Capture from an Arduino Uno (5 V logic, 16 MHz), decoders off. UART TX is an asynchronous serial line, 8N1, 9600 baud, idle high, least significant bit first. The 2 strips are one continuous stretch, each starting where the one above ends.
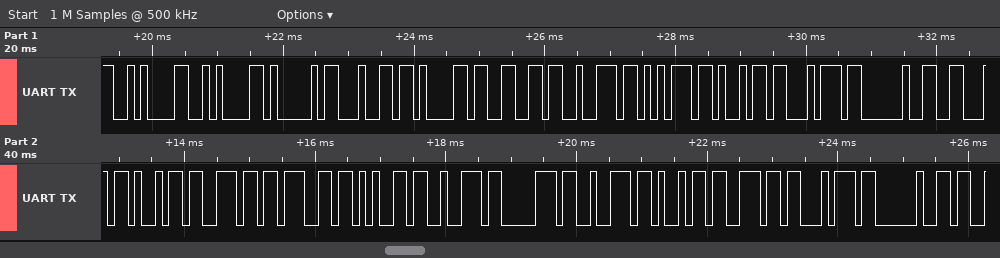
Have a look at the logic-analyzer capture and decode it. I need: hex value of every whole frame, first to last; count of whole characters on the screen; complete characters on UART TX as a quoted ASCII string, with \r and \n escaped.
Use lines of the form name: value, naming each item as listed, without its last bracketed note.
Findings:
hex value of every whole frame, first to last: 0A 0A 41 64 61 66 72 75 69 74 20 46 69 6E 67 65 72 70 72 69 6E 74 20
count of whole characters on the screen: 23
complete characters on UART TX as a quoted ASCII string, with \r and \n escaped: "\n\nAdafruit Fingerprint "
